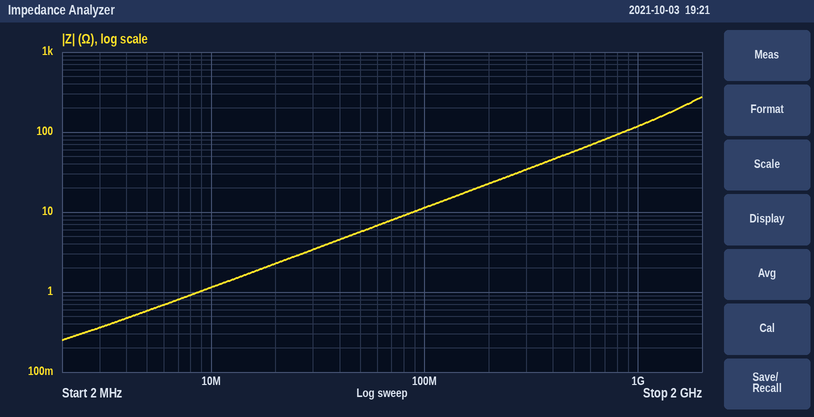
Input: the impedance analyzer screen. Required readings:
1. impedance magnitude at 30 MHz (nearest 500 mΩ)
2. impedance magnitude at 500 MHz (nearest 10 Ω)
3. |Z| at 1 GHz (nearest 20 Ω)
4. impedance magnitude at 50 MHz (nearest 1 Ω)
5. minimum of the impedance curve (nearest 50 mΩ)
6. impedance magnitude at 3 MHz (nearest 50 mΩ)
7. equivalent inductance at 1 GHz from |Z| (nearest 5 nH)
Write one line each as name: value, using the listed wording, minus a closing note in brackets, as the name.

impedance magnitude at 30 MHz: 3.5 Ω
impedance magnitude at 500 MHz: 60 Ω
|Z| at 1 GHz: 120 Ω
impedance magnitude at 50 MHz: 6 Ω
minimum of the impedance curve: 250 mΩ
impedance magnitude at 3 MHz: 350 mΩ
equivalent inductance at 1 GHz from |Z|: 20 nH
